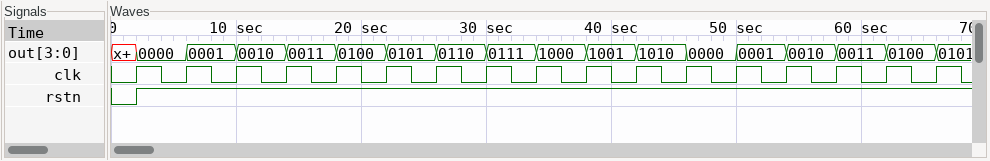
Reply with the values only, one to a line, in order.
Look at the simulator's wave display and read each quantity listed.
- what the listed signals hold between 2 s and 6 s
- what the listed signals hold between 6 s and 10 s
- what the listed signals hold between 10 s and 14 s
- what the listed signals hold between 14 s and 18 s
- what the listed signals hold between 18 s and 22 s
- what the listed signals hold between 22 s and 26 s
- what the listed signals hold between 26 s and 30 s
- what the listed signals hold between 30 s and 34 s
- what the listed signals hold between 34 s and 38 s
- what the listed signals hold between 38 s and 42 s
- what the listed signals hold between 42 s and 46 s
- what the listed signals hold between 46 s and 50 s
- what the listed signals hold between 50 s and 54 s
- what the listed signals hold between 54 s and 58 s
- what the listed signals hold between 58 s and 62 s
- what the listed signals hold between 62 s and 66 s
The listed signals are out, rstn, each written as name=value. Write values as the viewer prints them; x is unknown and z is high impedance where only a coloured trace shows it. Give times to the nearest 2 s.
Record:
out=0000, rstn=1
out=0001, rstn=1
out=0010, rstn=1
out=0011, rstn=1
out=0100, rstn=1
out=0101, rstn=1
out=0110, rstn=1
out=0111, rstn=1
out=1000, rstn=1
out=1001, rstn=1
out=1010, rstn=1
out=0000, rstn=1
out=0001, rstn=1
out=0010, rstn=1
out=0011, rstn=1
out=0100, rstn=1
